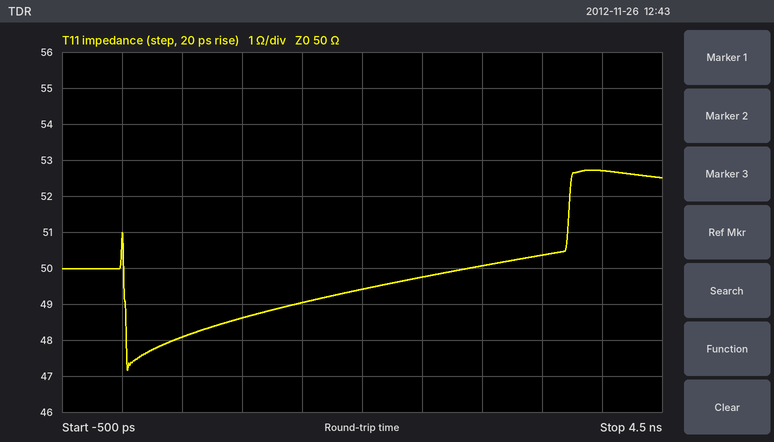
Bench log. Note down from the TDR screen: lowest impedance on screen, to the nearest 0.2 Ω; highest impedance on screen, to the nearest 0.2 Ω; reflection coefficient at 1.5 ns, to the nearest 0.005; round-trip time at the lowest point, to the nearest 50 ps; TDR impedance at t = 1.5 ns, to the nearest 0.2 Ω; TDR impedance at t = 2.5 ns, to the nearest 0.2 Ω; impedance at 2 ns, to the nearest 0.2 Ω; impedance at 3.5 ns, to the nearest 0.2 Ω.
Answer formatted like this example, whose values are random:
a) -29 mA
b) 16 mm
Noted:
a) 47.2 Ω
b) 52.8 Ω
c) -0.010
d) 50 ps
e) 49.0 Ω
f) 49.8 Ω
g) 49.4 Ω
h) 50.4 Ω
